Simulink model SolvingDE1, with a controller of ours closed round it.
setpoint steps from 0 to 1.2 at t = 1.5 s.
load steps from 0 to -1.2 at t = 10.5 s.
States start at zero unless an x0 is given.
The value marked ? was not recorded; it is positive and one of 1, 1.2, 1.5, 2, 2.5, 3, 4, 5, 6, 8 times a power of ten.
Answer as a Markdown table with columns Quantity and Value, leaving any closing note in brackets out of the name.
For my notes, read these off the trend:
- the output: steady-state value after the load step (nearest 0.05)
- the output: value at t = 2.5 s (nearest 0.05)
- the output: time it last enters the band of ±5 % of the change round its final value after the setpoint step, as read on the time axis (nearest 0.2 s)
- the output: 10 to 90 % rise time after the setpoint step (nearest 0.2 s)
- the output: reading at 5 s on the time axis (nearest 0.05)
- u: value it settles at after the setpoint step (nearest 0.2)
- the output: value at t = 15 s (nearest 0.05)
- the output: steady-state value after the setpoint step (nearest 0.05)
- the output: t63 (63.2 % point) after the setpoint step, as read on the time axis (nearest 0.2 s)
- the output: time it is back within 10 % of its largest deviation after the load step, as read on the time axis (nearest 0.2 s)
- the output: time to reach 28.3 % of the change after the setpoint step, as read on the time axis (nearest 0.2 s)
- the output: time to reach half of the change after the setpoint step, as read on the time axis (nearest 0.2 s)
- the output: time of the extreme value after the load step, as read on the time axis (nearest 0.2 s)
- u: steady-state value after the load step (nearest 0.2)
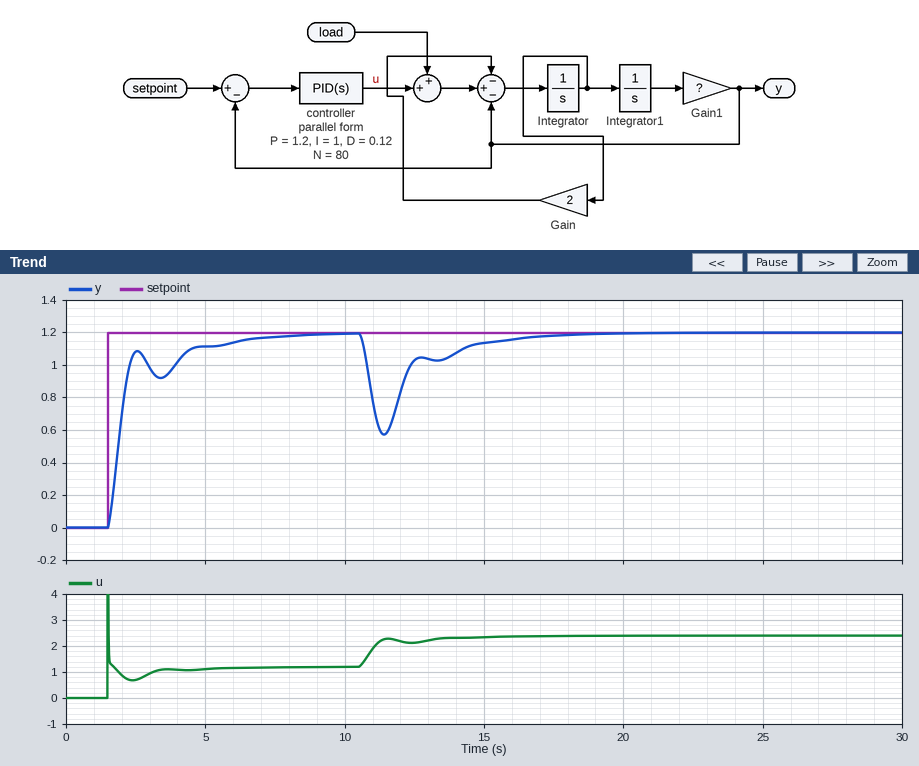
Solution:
| Quantity | Value |
|---|---|
| the output: steady-state value after the load step | 1.20 |
| the output: value at t = 2.5 s | 1.10 |
| the output: time it last enters the band of ±5 % of the change round its final value after the setpoint step, as read on the time axis | 6.0 s |
| the output: 10 to 90 % rise time after the setpoint step | 0.8 s |
| the output: reading at 5 s on the time axis | 1.10 |
| u: value it settles at after the setpoint step | 1.2 |
| the output: value at t = 15 s | 1.15 |
| the output: steady-state value after the setpoint step | 1.20 |
| the output: t63 (63.2 % point) after the setpoint step, as read on the time axis | 2.0 s |
| the output: time it is back within 10 % of its largest deviation after the load step, as read on the time axis | 15.2 s |
| the output: time to reach 28.3 % of the change after the setpoint step, as read on the time axis | 1.8 s |
| the output: time to reach half of the change after the setpoint step, as read on the time axis | 2.0 s |
| the output: time of the extreme value after the load step, as read on the time axis | 11.4 s |
| u: steady-state value after the load step | 2.4 |
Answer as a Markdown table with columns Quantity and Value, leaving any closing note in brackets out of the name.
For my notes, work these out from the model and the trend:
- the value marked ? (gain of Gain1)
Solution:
| Quantity | Value |
|---|---|
| the value marked ? | 5 |
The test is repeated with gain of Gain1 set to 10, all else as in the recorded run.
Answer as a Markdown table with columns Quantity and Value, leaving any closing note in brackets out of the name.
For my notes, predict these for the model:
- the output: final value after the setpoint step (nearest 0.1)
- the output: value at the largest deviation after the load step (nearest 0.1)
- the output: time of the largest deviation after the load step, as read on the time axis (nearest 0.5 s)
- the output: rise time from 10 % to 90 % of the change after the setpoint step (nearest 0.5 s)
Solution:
| Quantity | Value |
|---|---|
| the output: final value after the setpoint step | 1.2 |
| the output: value at the largest deviation after the load step | 0.5 |
| the output: time of the largest deviation after the load step, as read on the time axis | 11.0 s |
| the output: rise time from 10 % to 90 % of the change after the setpoint step | 3.0 s |
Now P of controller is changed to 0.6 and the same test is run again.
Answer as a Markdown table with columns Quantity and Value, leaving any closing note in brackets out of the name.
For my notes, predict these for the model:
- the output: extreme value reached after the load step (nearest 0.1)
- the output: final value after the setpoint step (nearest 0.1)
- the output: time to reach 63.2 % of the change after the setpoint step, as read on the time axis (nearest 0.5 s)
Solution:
| Quantity | Value |
|---|---|
| the output: extreme value reached after the load step | 0.4 |
| the output: final value after the setpoint step | 1.2 |
| the output: time to reach 63.2 % of the change after the setpoint step, as read on the time axis | 2.5 s |
